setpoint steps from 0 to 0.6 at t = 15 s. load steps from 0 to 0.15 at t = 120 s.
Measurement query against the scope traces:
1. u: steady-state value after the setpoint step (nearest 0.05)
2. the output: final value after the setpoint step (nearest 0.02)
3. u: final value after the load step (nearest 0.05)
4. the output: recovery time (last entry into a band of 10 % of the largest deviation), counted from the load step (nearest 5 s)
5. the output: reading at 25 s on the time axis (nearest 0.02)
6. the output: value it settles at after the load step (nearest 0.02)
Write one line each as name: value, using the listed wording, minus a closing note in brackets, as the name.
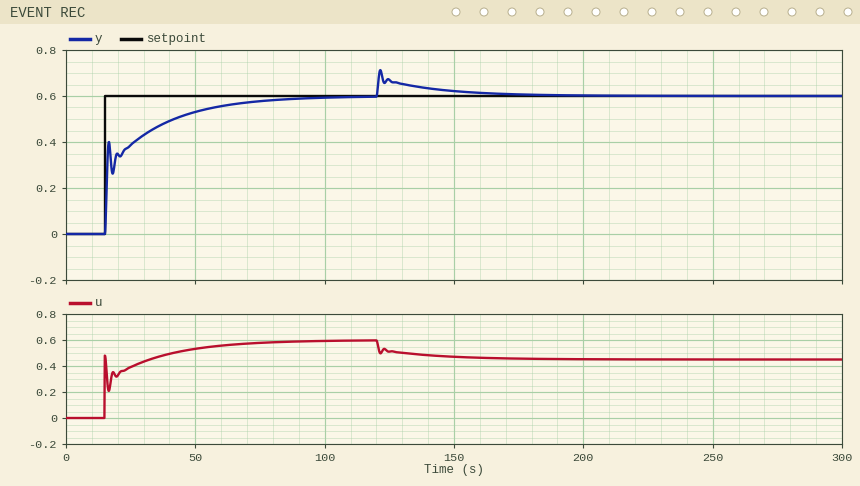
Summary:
u: steady-state value after the setpoint step: 0.60
the output: final value after the setpoint step: 0.60
u: final value after the load step: 0.45
the output: recovery time (last entry into a band of 10 % of the largest deviation), counted from the load step: 45 s
the output: reading at 25 s on the time axis: 0.38
the output: value it settles at after the load step: 0.60
